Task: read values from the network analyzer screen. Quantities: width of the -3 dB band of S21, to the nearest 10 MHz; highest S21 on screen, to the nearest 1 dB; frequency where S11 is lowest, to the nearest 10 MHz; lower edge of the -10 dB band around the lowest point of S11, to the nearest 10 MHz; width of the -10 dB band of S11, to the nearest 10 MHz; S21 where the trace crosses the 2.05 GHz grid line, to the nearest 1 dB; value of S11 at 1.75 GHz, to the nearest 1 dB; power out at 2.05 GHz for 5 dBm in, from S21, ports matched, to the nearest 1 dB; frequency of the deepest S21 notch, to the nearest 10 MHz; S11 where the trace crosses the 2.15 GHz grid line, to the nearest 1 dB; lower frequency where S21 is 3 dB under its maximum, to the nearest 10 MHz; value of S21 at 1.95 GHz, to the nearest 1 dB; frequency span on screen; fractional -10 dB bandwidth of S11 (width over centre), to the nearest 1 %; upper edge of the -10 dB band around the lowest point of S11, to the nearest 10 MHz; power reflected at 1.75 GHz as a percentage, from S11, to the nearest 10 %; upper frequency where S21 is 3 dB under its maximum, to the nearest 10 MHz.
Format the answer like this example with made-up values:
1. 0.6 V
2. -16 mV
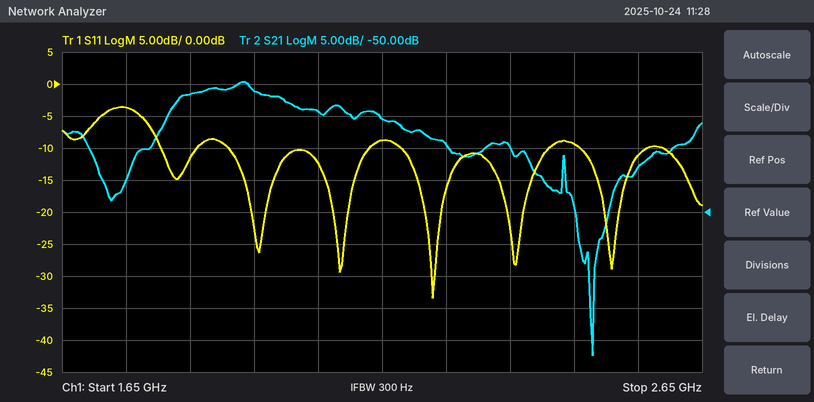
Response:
1. 170 MHz
2. -30 dB
3. 2.23 GHz
4. 2.18 GHz
5. 230 MHz
6. -34 dB
7. -4 dB
8. -29 dBm
9. 2.48 GHz
10. -9 dB
11. 1.83 GHz
12. -31 dB
13. 1 GHz
14. 10 %
15. 2.41 GHz
16. 40 %
17. 2.00 GHz
